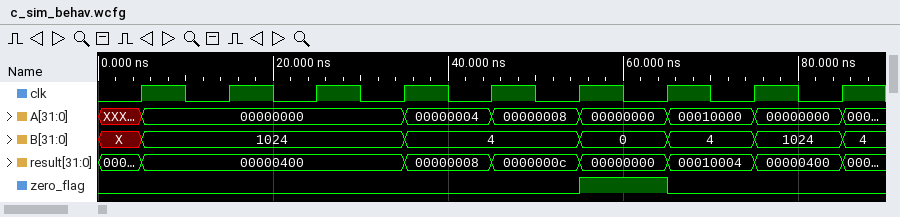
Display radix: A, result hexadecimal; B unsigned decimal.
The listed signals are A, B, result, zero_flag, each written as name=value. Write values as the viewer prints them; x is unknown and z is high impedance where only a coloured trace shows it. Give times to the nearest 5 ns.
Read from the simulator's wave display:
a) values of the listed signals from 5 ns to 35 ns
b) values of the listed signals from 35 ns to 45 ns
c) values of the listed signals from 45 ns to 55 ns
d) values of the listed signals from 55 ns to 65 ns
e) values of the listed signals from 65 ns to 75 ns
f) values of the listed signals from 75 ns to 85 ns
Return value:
A=00000000, B=1024, result=00000400, zero_flag=0
A=00000004, B=4, result=00000008, zero_flag=0
A=00000008, B=4, result=0000000c, zero_flag=0
A=00000000, B=0, result=00000000, zero_flag=1
A=00010000, B=4, result=00010004, zero_flag=0
A=00000000, B=1024, result=00000400, zero_flag=0
